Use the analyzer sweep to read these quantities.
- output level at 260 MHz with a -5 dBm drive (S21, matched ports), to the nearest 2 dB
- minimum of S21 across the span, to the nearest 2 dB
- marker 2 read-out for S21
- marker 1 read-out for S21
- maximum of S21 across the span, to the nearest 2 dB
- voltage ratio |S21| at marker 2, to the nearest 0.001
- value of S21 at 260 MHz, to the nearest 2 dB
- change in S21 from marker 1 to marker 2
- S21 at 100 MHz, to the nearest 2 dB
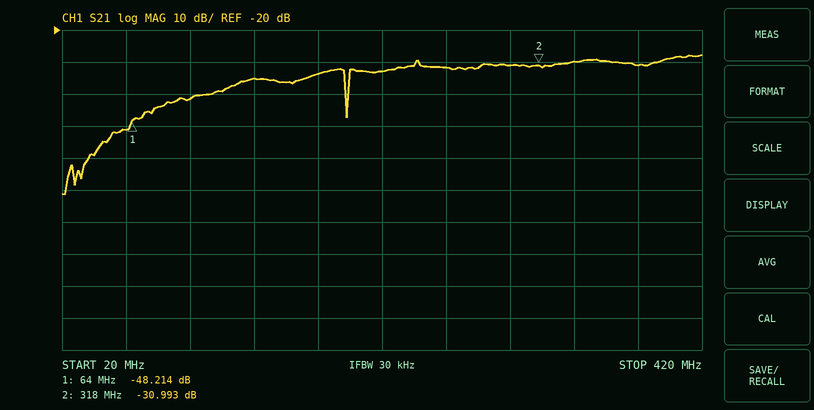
-36 dBm
-72 dB
-30.993 dB
-48.214 dB
-28 dB
0.028
-32 dB
17.221 dB
-42 dB
